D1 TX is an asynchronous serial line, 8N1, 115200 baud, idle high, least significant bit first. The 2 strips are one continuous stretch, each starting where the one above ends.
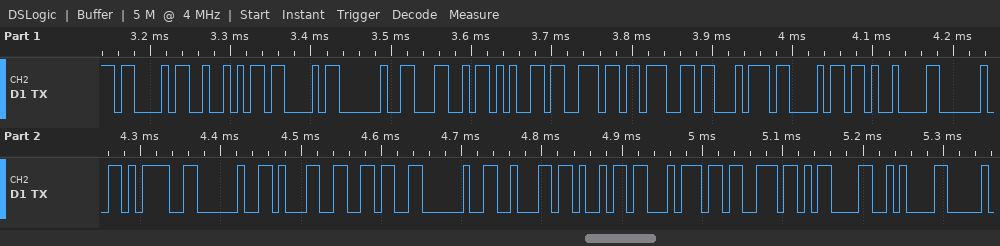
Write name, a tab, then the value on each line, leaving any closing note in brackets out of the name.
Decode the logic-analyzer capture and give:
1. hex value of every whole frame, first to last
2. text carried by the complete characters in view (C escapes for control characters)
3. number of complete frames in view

hex value of every whole frame, first to last	43 52 43 20 4C 65 6E 67 74 68 09 20 3D 20 31 36 20 62 69 74 73 0D 0A
text carried by the complete characters in view	"CRC Length\t = 16 bits\r\n"
number of complete frames in view	23
